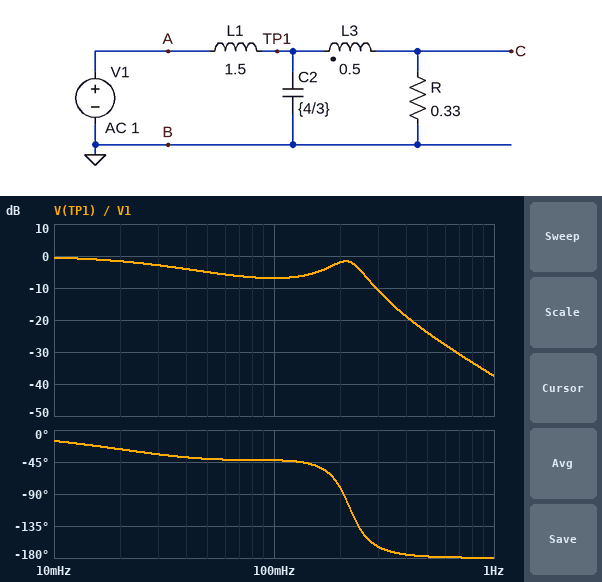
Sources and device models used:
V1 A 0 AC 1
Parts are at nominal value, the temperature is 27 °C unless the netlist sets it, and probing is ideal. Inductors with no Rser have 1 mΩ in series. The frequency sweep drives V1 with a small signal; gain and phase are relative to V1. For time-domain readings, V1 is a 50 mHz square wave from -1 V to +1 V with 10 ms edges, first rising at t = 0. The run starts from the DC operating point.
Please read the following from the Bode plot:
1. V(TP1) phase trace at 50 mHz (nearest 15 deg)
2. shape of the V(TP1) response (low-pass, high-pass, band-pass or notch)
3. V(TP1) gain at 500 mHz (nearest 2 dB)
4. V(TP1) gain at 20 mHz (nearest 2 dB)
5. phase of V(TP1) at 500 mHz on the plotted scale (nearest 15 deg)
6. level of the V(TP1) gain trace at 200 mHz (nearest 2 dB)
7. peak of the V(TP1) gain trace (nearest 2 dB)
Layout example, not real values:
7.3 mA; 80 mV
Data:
-45 deg; low-pass; -24 dB; -2 dB; -180 deg; -2 dB; 0 dB
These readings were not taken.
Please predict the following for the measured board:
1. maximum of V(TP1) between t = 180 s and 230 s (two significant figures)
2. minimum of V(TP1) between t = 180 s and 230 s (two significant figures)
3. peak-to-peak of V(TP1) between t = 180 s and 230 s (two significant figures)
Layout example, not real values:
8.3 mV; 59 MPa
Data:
730 mV; -730 mV; 1.5 V
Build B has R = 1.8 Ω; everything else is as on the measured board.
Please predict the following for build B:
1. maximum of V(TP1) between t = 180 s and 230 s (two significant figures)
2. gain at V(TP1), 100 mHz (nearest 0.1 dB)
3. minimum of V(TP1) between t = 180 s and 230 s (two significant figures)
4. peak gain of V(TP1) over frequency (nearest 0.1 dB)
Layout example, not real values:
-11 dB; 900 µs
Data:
1.7 V; 4.6 dB; -1.7 V; 4.8 dB
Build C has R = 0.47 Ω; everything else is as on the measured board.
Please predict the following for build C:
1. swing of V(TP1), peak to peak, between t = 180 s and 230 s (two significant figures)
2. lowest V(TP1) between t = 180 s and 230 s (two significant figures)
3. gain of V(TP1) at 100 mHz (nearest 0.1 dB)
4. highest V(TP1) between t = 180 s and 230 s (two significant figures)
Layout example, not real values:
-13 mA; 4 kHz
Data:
1.7 V; -870 mV; -5.1 dB; 870 mV
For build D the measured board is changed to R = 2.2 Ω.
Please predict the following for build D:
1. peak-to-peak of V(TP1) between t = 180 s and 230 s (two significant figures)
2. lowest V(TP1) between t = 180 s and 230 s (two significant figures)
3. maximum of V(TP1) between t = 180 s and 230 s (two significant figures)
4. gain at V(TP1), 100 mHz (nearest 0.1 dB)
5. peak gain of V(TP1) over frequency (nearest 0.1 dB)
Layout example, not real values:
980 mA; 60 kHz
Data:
3.6 V; -1.8 V; 1.8 V; 6.0 dB; 6.5 dB
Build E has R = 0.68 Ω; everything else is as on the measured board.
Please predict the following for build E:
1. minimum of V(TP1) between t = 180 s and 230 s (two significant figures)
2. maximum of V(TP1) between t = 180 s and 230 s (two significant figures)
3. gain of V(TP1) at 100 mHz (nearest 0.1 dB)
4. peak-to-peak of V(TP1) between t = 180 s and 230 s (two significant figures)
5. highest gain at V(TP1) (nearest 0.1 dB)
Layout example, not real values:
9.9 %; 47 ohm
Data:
-980 mV; 980 mV; -2.7 dB; 2.0 V; 0 dB
